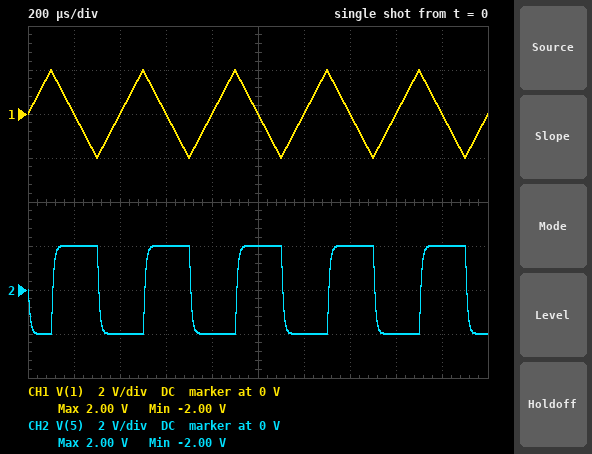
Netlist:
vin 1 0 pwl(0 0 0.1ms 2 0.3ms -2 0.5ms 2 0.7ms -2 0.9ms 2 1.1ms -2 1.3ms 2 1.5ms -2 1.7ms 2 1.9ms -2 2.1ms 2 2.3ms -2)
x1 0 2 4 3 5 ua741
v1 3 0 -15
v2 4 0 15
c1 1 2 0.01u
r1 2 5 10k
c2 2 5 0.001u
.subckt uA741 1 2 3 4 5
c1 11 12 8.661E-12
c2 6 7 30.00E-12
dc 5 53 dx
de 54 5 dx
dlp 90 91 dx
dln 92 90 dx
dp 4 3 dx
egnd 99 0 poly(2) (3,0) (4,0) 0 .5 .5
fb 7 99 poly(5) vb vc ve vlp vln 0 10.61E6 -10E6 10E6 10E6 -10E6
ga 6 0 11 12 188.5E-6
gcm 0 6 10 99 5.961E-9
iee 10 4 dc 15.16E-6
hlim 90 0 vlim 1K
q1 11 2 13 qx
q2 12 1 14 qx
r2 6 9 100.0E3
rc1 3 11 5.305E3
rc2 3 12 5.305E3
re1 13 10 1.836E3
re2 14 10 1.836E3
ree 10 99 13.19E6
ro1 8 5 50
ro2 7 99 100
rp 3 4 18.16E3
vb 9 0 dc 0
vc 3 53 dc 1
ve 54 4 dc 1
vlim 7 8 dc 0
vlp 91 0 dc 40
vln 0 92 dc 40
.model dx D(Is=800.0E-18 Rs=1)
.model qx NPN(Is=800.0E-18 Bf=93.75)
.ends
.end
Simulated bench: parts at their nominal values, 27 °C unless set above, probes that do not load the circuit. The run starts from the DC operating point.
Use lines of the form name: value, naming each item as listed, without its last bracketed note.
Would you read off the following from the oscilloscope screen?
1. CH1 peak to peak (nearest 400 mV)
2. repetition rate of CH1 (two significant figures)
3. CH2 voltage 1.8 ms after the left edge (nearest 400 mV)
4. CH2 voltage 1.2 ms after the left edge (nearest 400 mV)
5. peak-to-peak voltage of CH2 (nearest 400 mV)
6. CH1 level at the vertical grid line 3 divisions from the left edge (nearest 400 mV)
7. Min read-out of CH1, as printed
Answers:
CH1 peak to peak: 4.0 V
repetition rate of CH1: 2.5 kHz
CH2 voltage 1.8 ms after the left edge: 2.0 V
CH2 voltage 1.2 ms after the left edge: -2.0 V
peak-to-peak voltage of CH2: 4.0 V
CH1 level at the vertical grid line 3 divisions from the left edge: 0 V
Min read-out of CH1, as printed: -2.00 V
